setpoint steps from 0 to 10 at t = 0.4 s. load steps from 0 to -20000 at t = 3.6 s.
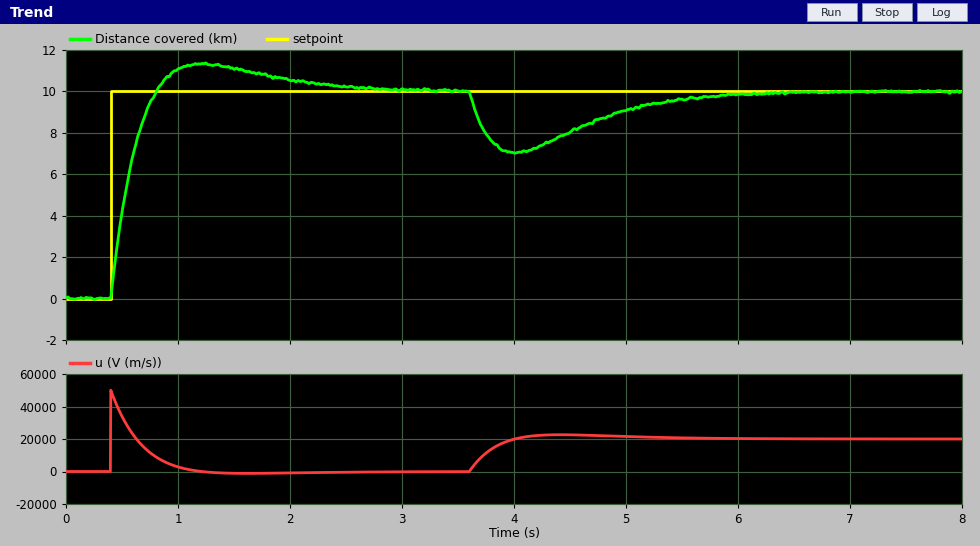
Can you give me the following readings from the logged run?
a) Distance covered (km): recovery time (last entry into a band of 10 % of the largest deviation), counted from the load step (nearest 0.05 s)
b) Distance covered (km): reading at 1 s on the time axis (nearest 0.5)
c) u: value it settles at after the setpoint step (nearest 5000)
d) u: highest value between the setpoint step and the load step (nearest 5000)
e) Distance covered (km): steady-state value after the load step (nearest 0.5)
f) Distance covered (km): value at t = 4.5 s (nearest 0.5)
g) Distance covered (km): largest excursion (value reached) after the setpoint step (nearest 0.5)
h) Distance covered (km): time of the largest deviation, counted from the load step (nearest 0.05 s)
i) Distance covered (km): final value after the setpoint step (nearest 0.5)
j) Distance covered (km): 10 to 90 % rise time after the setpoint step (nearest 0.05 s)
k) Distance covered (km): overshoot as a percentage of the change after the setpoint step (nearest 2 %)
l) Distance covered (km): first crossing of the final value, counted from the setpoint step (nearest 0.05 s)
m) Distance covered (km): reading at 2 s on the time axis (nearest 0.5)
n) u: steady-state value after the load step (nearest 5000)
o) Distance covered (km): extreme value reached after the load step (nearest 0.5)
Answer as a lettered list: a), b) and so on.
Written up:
a) 2.05 s
b) 11.0
c) 0
d) 50000
e) 10.0
f) 8.0
g) 11.5
h) 0.40 s
i) 10.0
j) 0.30 s
k) 14 %
l) 0.40 s
m) 10.5
n) 20000
o) 7.0
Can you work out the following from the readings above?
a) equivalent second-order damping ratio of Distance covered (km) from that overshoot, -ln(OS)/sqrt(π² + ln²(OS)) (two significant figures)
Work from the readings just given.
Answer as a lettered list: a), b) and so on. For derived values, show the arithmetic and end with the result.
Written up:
a) ln(0.14) = -1.966; 1.966 / sqrt(9.870 + 3.866) = 0.53
